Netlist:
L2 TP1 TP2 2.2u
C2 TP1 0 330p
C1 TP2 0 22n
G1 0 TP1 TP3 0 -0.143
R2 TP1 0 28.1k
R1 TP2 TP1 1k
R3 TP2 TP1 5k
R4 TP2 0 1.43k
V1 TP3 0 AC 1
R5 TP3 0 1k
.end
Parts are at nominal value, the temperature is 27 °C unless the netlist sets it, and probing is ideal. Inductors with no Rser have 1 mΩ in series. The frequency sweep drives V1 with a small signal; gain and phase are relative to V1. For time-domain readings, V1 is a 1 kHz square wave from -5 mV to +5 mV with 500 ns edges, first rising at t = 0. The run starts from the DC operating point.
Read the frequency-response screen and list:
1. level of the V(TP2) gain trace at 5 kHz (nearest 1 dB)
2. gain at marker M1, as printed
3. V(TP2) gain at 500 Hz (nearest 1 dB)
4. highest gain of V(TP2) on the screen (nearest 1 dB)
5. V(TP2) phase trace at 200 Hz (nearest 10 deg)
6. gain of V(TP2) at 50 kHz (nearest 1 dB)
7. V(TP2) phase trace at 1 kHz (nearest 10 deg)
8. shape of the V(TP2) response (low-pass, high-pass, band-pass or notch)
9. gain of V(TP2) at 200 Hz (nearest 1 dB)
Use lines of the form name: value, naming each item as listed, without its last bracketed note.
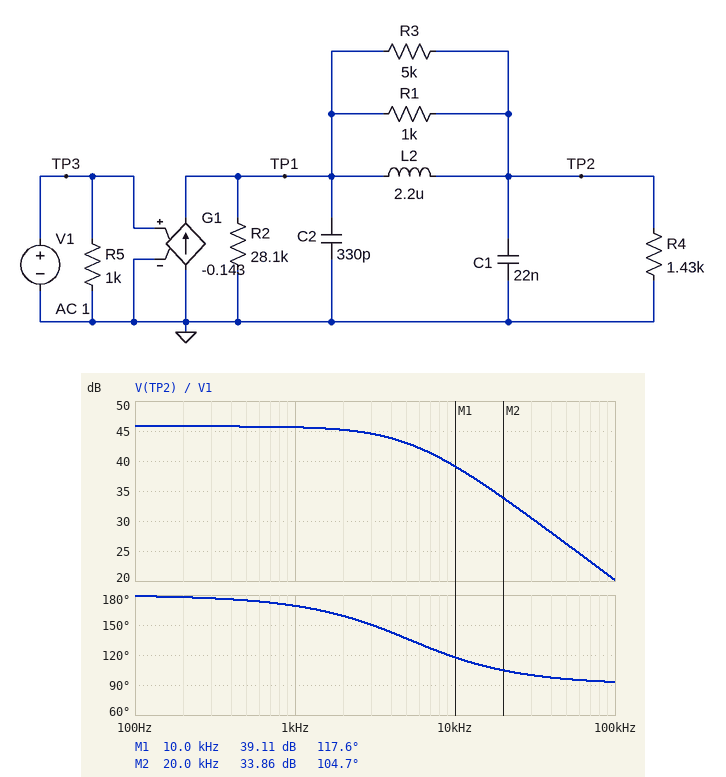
level of the V(TP2) gain trace at 5 kHz: 43 dB
gain at marker M1, as printed: 39.11 dB
V(TP2) gain at 500 Hz: 46 dB
highest gain of V(TP2) on the screen: 46 dB
V(TP2) phase trace at 200 Hz: 180 deg
gain of V(TP2) at 50 kHz: 26 dB
V(TP2) phase trace at 1 kHz: 170 deg
shape of the V(TP2) response: low-pass
gain of V(TP2) at 200 Hz: 46 dB
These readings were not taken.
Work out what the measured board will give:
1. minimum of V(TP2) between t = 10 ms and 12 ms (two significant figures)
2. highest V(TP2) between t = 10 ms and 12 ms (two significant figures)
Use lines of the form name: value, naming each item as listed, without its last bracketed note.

minimum of V(TP2) between t = 10 ms and 12 ms: -970 mV
highest V(TP2) between t = 10 ms and 12 ms: 970 mV
